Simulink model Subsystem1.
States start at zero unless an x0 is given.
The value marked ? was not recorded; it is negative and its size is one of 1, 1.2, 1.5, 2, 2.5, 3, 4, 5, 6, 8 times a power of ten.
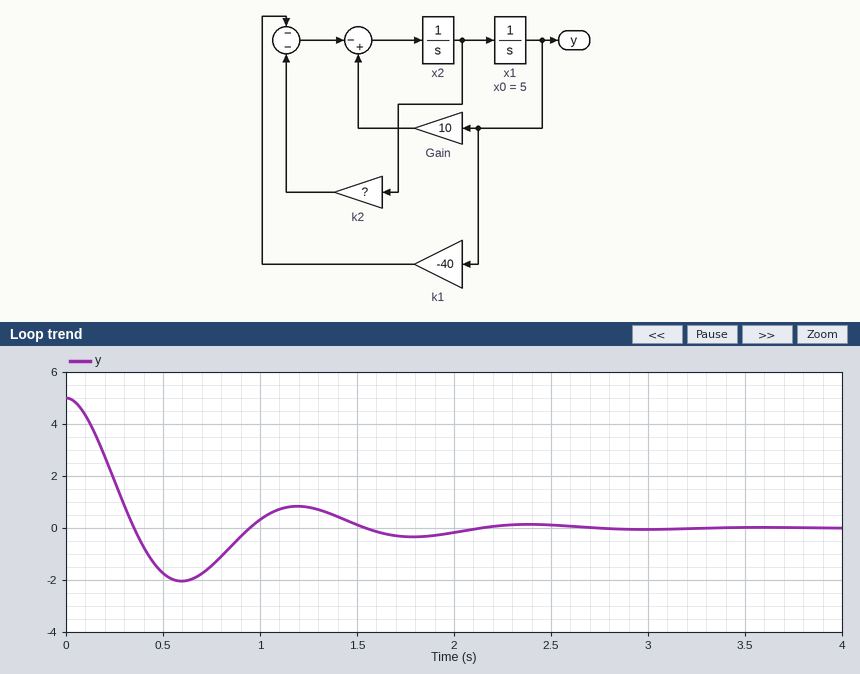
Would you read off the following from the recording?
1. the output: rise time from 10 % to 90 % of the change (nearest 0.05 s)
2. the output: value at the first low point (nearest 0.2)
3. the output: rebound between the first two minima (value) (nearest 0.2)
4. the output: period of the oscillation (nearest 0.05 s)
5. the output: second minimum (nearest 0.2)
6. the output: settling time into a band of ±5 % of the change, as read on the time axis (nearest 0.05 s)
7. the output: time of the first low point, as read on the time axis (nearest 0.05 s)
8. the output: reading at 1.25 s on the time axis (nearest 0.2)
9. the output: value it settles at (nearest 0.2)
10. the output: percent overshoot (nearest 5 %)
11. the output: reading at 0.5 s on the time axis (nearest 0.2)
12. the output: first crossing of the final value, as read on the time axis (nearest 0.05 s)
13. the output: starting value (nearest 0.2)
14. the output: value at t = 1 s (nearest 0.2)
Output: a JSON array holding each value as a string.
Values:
["0.25 s", "-2.0", "0.8", "1.20 s", "-0.4", "1.95 s", "0.60 s", "0.8", "0.0", "40 %", "-1.8", "0.35 s", "5.0", "0.4"]
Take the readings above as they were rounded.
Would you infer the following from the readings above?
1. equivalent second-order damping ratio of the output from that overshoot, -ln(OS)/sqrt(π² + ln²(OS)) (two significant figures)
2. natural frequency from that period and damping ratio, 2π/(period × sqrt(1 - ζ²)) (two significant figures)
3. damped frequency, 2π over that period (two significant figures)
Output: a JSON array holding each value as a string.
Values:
["0.28", "5.5 rad/s", "5.2 rad/s"]
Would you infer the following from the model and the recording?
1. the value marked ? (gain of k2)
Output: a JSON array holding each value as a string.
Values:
["-3"]
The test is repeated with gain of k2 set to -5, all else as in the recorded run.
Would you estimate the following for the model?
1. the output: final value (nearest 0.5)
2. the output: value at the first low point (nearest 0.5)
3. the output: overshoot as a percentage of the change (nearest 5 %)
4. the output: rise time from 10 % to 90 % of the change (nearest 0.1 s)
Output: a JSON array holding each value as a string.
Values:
["0.0", "-1.0", "20 %", "0.3 s"]
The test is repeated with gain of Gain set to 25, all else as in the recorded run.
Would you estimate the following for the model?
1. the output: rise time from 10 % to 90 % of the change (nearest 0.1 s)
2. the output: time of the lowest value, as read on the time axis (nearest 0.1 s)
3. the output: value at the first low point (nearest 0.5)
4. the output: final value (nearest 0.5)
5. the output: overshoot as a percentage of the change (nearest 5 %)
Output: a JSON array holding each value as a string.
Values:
["0.4 s", "0.9 s", "-1.5", "0.0", "25 %"]
